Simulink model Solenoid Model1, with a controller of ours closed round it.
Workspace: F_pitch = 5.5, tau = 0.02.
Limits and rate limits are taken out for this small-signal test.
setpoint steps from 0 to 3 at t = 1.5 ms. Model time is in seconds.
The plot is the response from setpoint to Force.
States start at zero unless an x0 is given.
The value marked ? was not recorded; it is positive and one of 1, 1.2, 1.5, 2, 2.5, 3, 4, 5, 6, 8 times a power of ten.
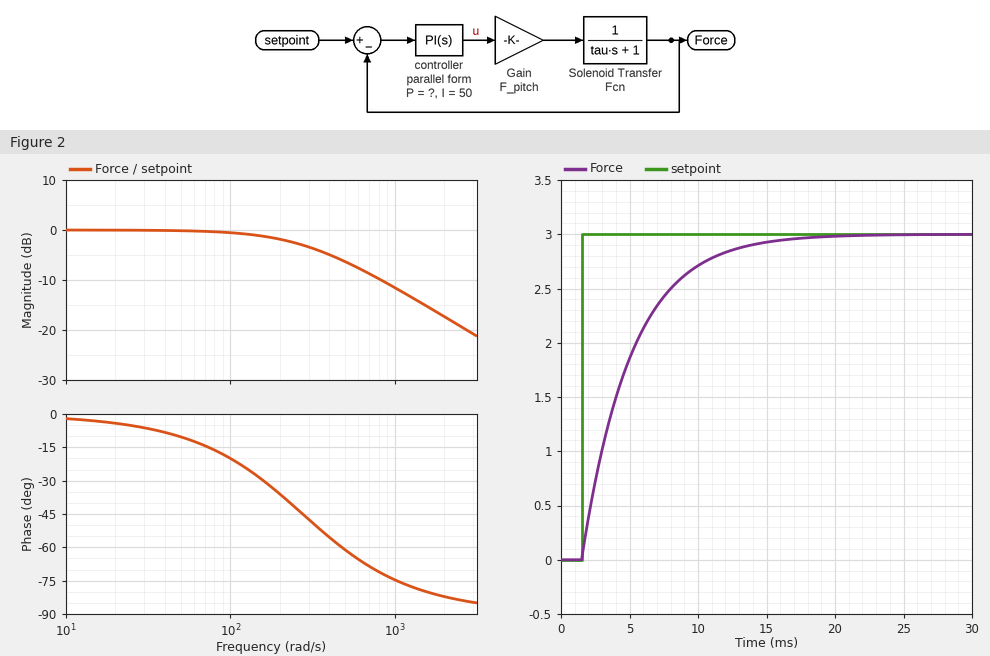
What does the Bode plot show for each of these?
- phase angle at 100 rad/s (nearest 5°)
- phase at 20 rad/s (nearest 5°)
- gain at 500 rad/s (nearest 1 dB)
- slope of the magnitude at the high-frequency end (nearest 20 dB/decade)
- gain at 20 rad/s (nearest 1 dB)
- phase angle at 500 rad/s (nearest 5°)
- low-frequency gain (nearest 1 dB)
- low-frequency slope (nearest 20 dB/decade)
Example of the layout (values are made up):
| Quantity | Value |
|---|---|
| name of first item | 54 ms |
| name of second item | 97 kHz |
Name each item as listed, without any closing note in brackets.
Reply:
| Quantity | Value |
|---|---|
| phase angle at 100 rad/s | -20° |
| phase at 20 rad/s | -5° |
| gain at 500 rad/s | -6 dB |
| slope of the magnitude at the high-frequency end | -20 dB/decade |
| gain at 20 rad/s | 0 dB |
| phase angle at 500 rad/s | -60° |
| low-frequency gain | 0 dB |
| low-frequency slope | 0 dB/decade |
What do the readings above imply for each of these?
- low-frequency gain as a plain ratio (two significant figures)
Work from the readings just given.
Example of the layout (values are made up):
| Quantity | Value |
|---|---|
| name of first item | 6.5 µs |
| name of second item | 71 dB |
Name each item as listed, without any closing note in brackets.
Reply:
| Quantity | Value |
|---|---|
| low-frequency gain as a plain ratio | 1.0 |
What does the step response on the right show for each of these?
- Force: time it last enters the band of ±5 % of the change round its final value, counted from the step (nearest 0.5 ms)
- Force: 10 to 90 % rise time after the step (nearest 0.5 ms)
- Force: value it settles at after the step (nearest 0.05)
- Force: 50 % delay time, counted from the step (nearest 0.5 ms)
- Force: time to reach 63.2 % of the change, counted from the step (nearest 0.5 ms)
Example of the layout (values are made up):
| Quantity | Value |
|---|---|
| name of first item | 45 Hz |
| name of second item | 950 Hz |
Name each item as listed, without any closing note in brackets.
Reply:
| Quantity | Value |
|---|---|
| Force: time it last enters the band of ±5 % of the change round its final value, counted from the step | 11.0 ms |
| Force: 10 to 90 % rise time after the step | 8.0 ms |
| Force: value it settles at after the step | 3.00 |
| Force: 50 % delay time, counted from the step | 2.5 ms |
| Force: time to reach 63.2 % of the change, counted from the step | 3.5 ms |
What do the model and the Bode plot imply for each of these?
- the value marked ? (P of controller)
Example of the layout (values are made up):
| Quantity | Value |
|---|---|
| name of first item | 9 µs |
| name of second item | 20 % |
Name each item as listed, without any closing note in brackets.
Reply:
| Quantity | Value |
|---|---|
| the value marked ? | 1 |
